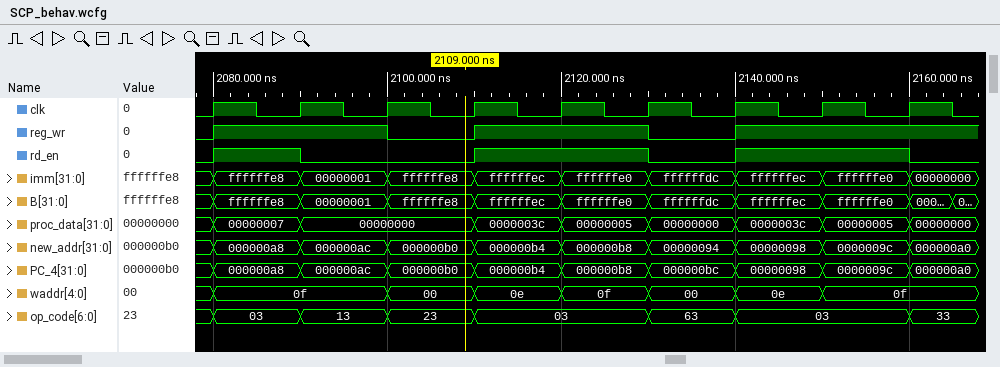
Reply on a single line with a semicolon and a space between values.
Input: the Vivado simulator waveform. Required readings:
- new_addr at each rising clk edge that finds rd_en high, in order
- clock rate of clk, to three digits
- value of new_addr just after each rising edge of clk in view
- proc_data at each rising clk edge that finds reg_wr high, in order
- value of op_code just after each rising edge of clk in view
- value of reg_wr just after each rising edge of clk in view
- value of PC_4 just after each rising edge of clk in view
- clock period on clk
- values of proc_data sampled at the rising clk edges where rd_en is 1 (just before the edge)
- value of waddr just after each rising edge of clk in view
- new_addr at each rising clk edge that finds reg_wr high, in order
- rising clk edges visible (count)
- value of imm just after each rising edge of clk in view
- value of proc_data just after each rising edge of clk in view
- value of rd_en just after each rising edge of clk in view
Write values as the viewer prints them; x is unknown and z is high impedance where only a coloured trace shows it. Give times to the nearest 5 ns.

000000a8, 000000b4, 000000b8, 00000098, 0000009c; 100 MHz; 000000a8, 000000ac, 000000b0, 000000b4, 000000b8, 00000094, 00000098, 0000009c, 000000a0; 00000007, 00000000, 0000003c, 00000005, 0000003c, 00000005; 03, 13, 23, 03, 03, 63, 03, 03, 33; 1 1 0 1 1 0 1 1 1; 000000a8, 000000ac, 000000b0, 000000b4, 000000b8, 000000bc, 00000098, 0000009c, 000000a0; 10 ns; 00000007, 0000003c, 00000005, 0000003c, 00000005; 0f, 0f, 00, 0e, 0f, 00, 0e, 0f, 0f; 000000a8, 000000ac, 000000b4, 000000b8, 00000098, 0000009c; 9; ffffffe8, 00000001, ffffffe8, ffffffec, ffffffe0, ffffffdc, ffffffec, ffffffe0, 00000000; 00000007, 00000000, 00000000, 0000003c, 00000005, 00000000, 0000003c, 00000005, 00000000; 1 0 0 1 1 0 1 1 0
